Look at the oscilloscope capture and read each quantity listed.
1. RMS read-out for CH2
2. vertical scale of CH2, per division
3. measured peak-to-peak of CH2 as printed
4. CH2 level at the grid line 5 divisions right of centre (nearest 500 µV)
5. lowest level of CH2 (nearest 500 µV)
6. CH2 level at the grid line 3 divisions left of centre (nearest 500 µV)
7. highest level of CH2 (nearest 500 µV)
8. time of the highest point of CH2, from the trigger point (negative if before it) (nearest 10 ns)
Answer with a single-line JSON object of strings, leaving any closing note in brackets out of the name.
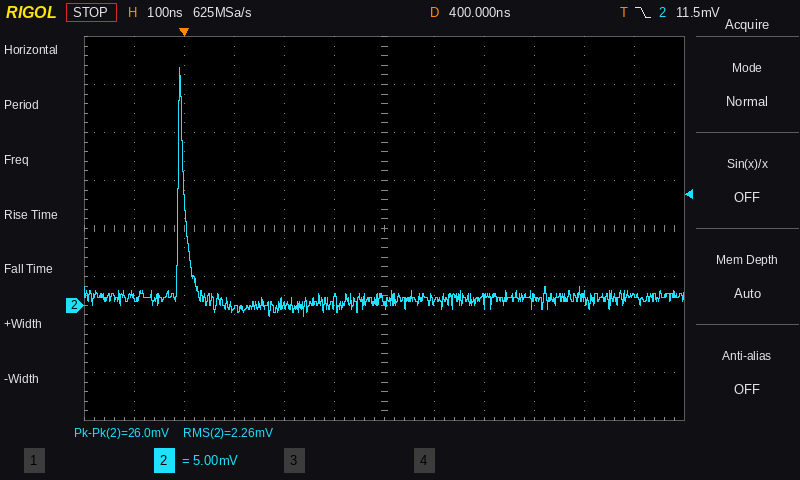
{"RMS read-out for CH2": "2.26 mV", "vertical scale of CH2, per division": "5 mV", "measured peak-to-peak of CH2 as printed": "26.0 mV", "CH2 level at the grid line 5 divisions right of centre": "1.0 mV", "lowest level of CH2": "-1.0 mV", "CH2 level at the grid line 3 divisions left of centre": "-500 µV", "highest level of CH2": "25.0 mV", "time of the highest point of CH2, from the trigger point (negative if before it)": "-10 ns"}
